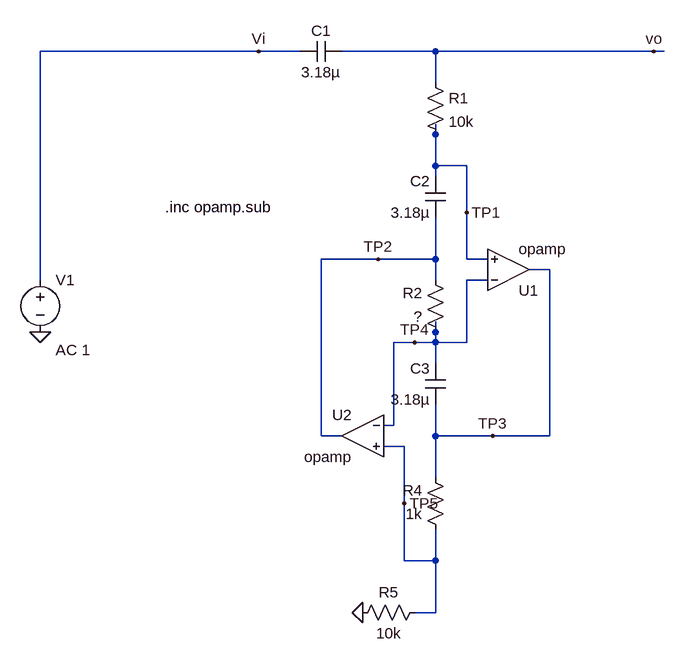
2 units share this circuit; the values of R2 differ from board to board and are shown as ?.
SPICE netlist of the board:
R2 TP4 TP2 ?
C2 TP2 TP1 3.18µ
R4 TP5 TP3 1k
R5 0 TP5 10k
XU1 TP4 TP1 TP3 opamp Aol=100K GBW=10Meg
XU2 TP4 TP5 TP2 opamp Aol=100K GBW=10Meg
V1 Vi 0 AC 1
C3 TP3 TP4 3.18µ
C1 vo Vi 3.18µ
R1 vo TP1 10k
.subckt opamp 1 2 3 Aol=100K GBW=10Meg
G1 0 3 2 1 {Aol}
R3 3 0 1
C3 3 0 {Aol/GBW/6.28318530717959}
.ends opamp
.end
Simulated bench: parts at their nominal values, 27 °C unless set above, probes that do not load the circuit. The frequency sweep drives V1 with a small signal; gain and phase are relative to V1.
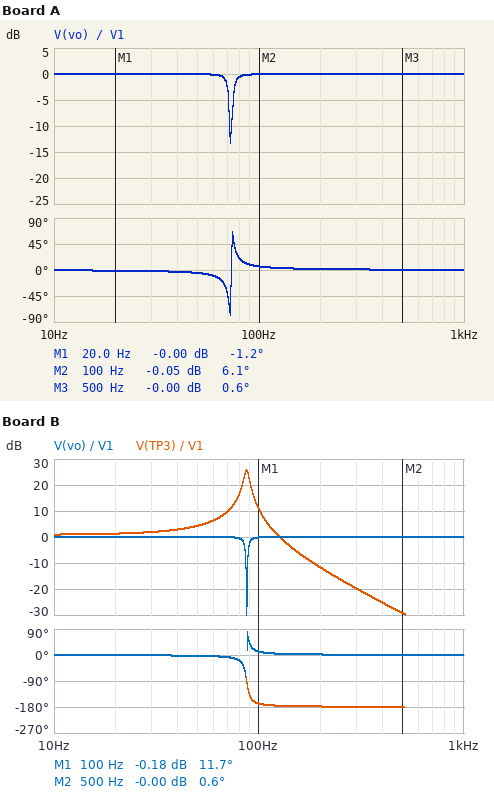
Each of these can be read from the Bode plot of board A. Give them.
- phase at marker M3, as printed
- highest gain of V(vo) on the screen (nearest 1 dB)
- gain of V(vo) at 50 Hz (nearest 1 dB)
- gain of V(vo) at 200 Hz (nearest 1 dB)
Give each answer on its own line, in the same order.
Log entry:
0.6 deg
0 dB
0 dB
0 dB
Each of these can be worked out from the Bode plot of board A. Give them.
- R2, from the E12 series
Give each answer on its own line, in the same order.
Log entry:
470 Ω
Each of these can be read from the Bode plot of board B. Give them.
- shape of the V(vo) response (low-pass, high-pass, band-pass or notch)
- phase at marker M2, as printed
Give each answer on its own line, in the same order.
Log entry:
notch
0.6 deg
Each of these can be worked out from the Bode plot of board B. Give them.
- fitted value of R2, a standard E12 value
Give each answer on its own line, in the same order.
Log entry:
330 Ω
